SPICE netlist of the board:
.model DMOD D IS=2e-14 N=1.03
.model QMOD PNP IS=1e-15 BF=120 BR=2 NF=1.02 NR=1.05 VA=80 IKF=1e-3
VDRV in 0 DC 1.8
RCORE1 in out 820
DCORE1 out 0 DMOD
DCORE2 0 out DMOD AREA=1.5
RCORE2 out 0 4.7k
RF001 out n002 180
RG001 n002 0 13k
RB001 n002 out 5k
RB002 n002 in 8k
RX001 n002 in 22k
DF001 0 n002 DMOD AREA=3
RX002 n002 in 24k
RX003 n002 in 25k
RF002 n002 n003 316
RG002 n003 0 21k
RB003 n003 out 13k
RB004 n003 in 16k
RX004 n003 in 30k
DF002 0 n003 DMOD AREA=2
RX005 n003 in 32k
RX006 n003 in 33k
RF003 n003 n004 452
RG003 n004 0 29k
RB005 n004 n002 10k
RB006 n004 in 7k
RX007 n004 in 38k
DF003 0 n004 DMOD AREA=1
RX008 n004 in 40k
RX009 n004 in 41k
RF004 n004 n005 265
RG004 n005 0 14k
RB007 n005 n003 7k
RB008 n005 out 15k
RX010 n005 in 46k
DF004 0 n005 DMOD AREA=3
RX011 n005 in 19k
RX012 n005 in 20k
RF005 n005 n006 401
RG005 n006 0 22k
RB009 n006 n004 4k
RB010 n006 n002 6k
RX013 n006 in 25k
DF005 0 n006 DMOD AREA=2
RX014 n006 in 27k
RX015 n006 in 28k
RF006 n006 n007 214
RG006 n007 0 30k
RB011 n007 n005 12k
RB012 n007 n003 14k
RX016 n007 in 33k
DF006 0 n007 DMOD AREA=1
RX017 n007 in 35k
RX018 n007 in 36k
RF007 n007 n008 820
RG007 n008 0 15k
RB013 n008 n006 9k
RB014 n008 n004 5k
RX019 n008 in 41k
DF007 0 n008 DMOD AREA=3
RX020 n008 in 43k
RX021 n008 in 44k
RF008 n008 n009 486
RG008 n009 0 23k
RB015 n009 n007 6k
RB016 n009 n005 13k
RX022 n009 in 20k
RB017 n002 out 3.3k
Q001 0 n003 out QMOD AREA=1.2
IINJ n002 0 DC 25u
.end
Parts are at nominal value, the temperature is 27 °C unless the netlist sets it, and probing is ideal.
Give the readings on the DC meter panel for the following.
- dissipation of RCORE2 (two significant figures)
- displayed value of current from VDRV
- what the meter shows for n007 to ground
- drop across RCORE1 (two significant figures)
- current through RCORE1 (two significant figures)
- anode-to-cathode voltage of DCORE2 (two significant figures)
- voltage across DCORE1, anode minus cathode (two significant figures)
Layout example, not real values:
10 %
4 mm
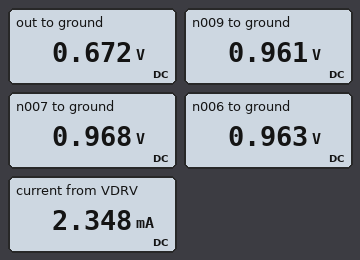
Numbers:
96 µW
2.348 mA
0.968 V
1.1 V
1.4 mA
-670 mV
670 mV
